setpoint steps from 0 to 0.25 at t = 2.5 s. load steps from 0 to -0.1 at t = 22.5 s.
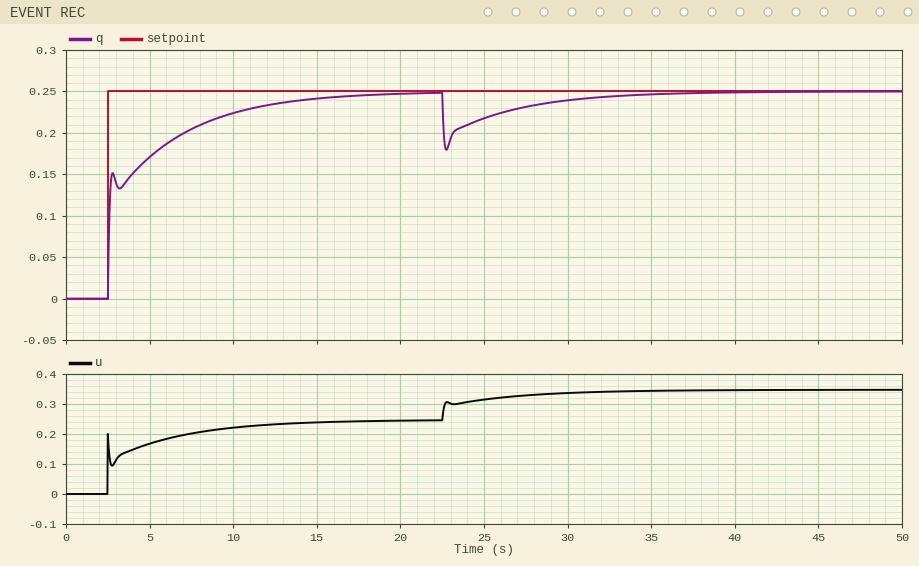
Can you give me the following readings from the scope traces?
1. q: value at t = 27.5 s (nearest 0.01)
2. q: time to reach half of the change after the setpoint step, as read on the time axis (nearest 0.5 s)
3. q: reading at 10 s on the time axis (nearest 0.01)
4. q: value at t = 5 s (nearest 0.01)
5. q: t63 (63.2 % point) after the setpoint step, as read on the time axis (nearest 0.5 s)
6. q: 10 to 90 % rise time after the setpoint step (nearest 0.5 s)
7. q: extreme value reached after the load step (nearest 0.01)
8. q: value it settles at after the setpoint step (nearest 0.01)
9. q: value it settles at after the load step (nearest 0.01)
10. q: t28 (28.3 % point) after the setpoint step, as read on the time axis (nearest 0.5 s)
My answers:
0.23
2.5 s
0.22
0.17
4.5 s
7.5 s
0.18
0.25
0.25
2.5 s
